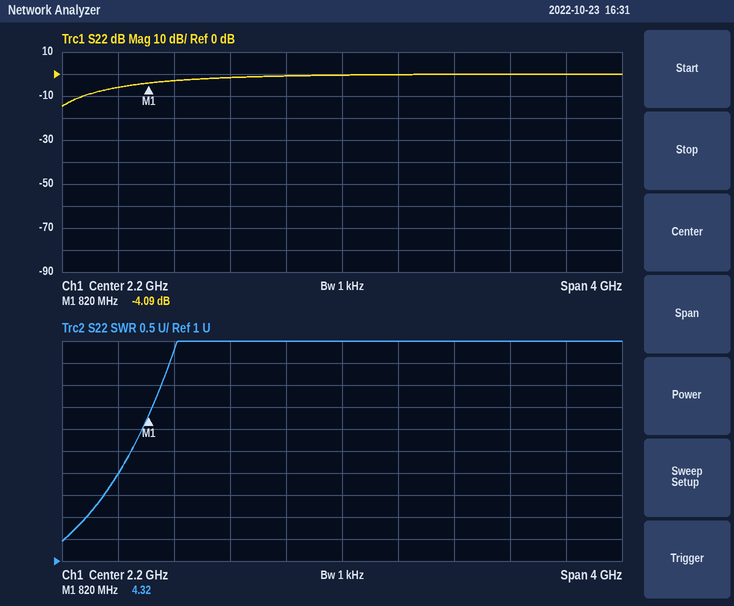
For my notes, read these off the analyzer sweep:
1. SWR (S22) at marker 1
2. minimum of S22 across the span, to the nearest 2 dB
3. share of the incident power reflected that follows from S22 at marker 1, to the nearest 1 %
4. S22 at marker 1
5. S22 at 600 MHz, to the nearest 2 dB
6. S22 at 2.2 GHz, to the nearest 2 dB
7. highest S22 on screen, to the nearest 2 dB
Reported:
4.32
-14 dB
39 %
-4.09 dB
-6 dB
0 dB
0 dB
